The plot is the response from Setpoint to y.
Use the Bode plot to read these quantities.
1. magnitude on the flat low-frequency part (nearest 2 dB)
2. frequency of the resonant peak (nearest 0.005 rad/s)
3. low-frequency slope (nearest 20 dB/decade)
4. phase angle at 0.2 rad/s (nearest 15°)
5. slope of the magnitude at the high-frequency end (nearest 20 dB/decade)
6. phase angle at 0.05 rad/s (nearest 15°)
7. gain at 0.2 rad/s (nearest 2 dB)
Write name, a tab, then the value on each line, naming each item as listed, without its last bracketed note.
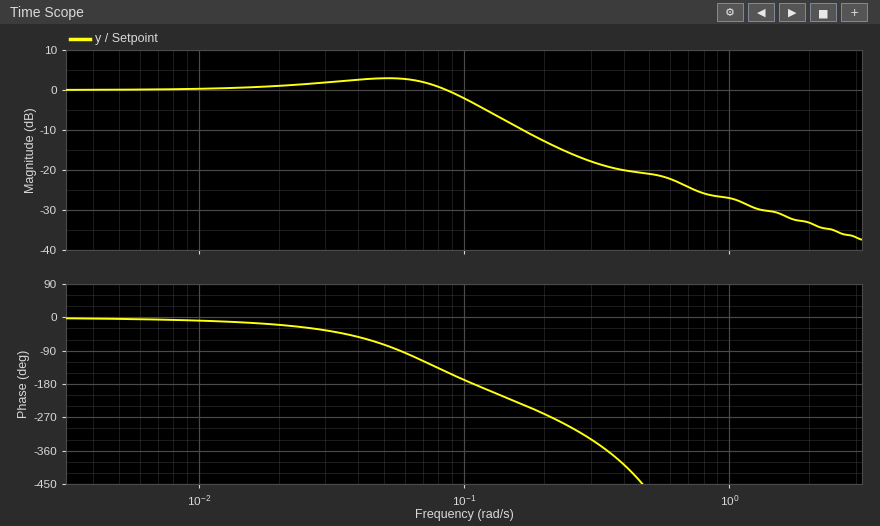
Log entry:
magnitude on the flat low-frequency part	0 dB
frequency of the resonant peak	0.050 rad/s
low-frequency slope	0 dB/decade
phase angle at 0.2 rad/s	-255°
slope of the magnitude at the high-frequency end	-20 dB/decade
phase angle at 0.05 rad/s	-75°
gain at 0.2 rad/s	-12 dB
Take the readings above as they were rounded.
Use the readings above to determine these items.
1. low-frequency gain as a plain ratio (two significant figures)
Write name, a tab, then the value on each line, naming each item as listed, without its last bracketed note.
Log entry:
low-frequency gain as a plain ratio	1.0
